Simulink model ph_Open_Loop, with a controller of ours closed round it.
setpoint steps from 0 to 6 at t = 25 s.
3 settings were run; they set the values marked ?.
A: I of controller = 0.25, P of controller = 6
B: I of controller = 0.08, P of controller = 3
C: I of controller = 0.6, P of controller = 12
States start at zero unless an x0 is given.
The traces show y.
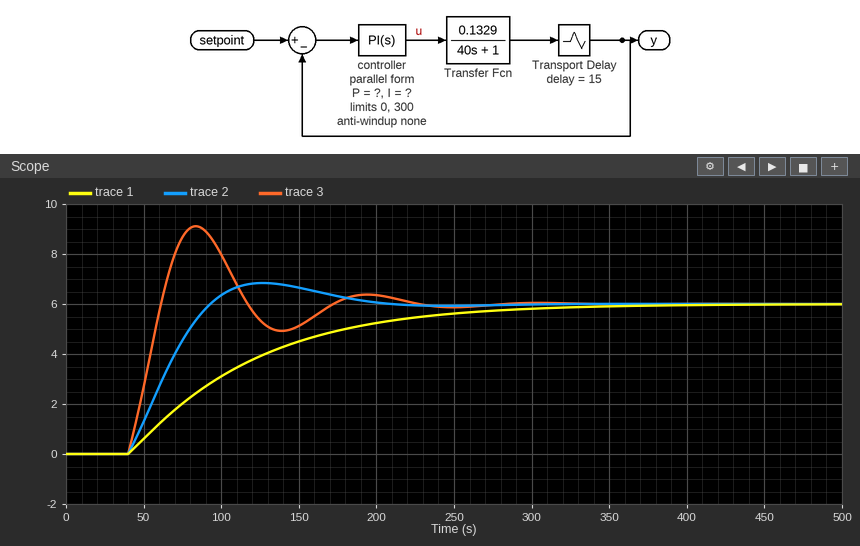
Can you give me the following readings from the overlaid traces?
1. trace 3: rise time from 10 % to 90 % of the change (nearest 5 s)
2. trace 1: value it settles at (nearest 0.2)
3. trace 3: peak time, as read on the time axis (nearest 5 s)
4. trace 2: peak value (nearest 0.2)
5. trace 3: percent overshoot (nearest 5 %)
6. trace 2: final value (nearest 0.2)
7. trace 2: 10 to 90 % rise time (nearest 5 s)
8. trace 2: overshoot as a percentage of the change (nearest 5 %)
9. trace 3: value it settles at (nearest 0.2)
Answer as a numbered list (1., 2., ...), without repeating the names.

1. 15 s
2. 6.0
3. 85 s
4. 6.8
5. 50 %
6. 6.0
7. 40 s
8. 15 %
9. 6.0
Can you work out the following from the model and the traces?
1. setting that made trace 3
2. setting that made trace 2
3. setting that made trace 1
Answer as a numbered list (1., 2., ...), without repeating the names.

1. C
2. A
3. B
